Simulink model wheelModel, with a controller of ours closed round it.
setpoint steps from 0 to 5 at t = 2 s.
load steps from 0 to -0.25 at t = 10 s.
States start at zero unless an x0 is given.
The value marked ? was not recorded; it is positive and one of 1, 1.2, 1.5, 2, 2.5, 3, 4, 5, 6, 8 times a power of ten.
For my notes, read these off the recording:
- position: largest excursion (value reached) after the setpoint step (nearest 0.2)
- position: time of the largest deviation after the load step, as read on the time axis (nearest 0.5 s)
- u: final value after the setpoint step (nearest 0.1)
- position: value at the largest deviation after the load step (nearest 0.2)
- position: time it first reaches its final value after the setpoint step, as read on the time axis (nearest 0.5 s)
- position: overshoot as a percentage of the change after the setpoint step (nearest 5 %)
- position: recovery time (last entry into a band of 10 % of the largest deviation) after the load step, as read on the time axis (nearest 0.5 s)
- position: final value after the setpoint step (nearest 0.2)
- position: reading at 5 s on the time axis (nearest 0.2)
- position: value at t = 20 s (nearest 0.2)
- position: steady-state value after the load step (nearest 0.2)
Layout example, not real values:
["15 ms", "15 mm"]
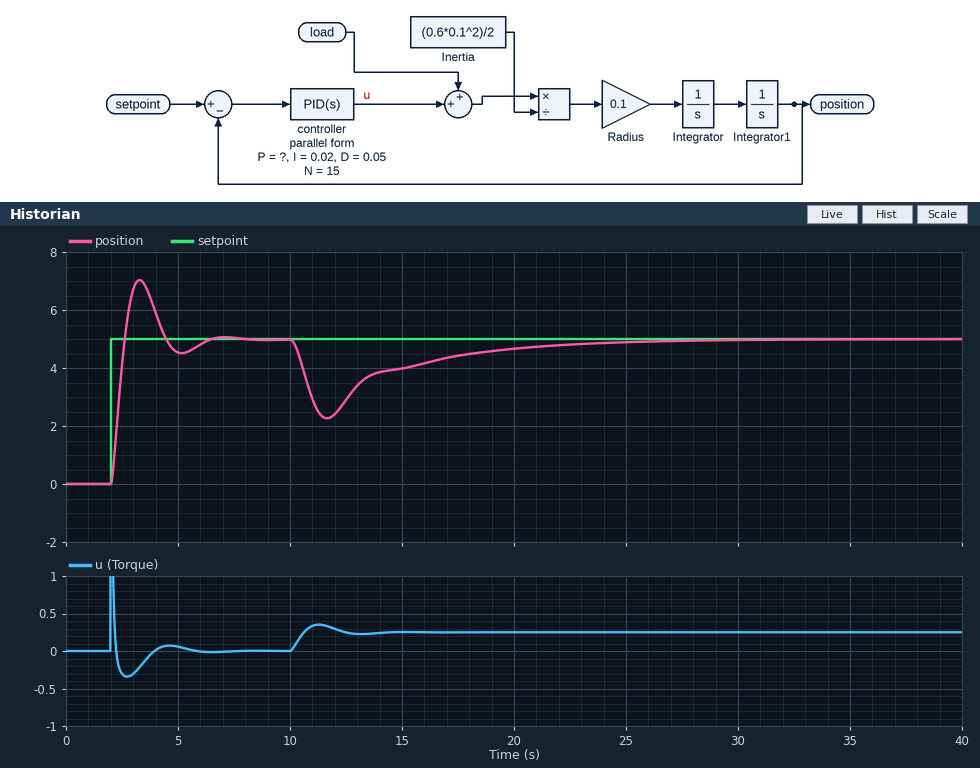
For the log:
["7.0", "11.5 s", "0.0", "2.2", "2.5 s", "40 %", "21.0 s", "5.0", "4.6", "4.6", "5.0"]
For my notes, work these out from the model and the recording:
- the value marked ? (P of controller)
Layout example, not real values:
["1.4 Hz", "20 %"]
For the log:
["0.1"]
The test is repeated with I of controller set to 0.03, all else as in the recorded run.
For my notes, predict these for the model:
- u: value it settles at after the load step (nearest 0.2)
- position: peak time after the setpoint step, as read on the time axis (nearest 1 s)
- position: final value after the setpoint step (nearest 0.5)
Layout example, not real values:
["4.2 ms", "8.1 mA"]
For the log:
["0.2", "3 s", "5.0"]
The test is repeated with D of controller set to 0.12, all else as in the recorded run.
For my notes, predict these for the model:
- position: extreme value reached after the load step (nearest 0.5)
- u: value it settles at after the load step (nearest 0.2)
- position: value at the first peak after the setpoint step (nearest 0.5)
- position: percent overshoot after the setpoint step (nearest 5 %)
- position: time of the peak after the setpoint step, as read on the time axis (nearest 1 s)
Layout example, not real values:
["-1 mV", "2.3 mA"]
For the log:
["3.0", "0.2", "6.0", "15 %", "3 s"]
